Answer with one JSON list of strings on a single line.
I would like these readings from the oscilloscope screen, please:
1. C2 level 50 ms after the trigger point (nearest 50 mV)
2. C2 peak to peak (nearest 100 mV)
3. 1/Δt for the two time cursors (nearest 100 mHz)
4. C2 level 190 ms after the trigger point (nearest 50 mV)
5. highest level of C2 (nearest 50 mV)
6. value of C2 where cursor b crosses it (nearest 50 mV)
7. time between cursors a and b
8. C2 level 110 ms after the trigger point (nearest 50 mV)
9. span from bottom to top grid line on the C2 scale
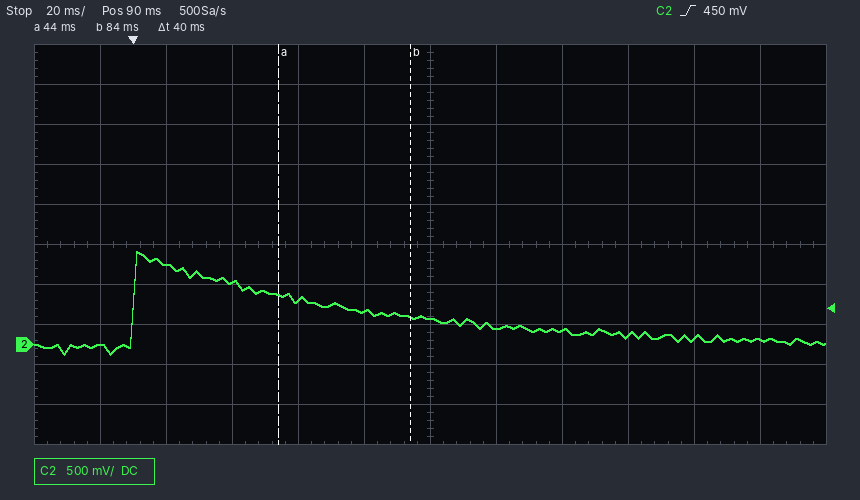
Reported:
["550 mV", "1.30 V", "25.0 Hz", "50 mV", "1.15 V", "350 mV", "40 ms", "200 mV", "5 V"]
